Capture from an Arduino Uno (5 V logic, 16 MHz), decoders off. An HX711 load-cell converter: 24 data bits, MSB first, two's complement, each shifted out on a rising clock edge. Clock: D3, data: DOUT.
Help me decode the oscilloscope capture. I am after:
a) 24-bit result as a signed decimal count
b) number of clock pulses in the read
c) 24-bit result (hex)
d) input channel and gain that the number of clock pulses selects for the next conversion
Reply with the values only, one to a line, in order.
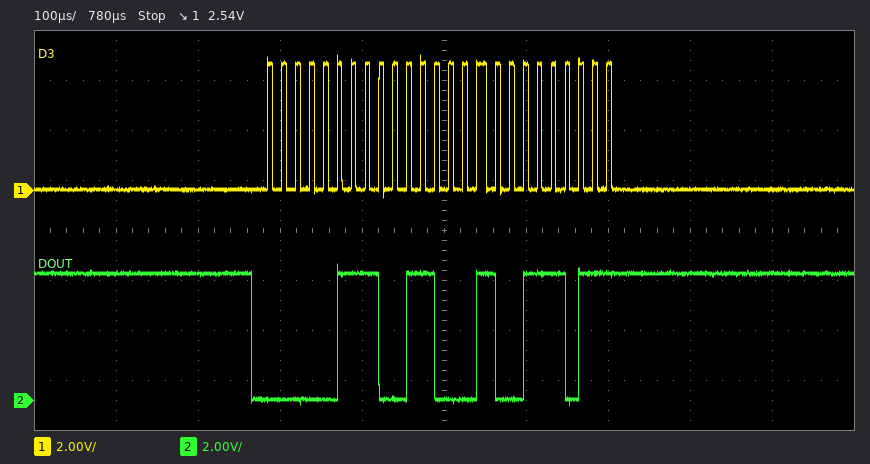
471355
25
0x07313B
channel A, gain 128
